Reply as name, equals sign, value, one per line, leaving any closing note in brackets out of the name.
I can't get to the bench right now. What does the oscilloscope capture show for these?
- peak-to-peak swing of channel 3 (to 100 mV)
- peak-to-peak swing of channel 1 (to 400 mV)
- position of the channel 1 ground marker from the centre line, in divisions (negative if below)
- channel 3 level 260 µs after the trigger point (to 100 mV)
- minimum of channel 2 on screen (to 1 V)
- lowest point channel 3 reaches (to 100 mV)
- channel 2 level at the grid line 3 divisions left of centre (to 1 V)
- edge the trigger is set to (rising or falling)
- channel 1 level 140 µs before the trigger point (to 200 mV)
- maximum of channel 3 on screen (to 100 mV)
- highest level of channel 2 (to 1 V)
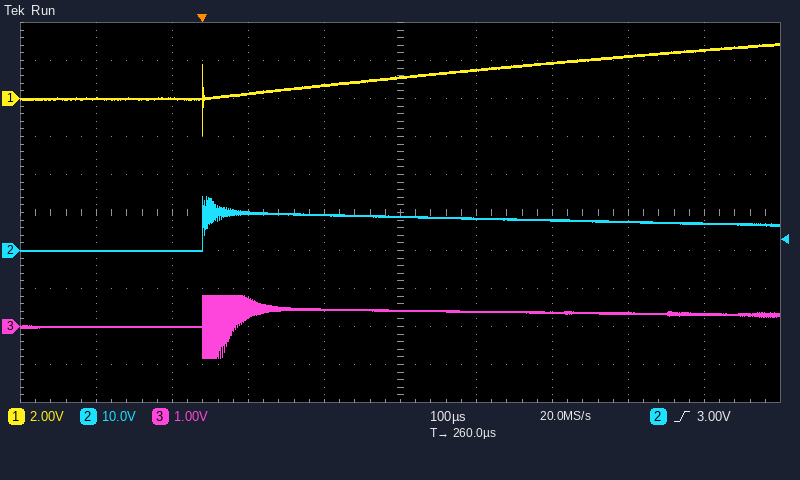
peak-to-peak swing of channel 3 = 1.6 V
peak-to-peak swing of channel 1 = 4.8 V
position of the channel 1 ground marker from the centre line, in divisions = +3.0 div
channel 3 level 260 µs after the trigger point = 400 mV
minimum of channel 2 on screen = 0 V
lowest point channel 3 reaches = -800 mV
channel 2 level at the grid line 3 divisions left of centre = 0 V
edge the trigger is set to = rising
channel 1 level 140 µs before the trigger point = 0.0 V
maximum of channel 3 on screen = 800 mV
highest level of channel 2 = 14 V
